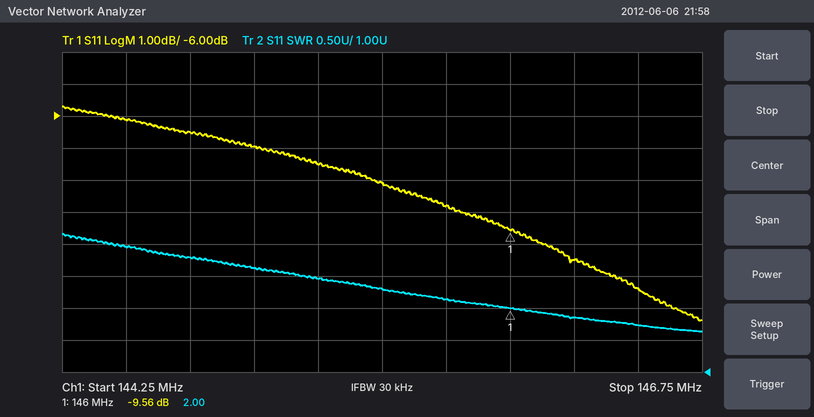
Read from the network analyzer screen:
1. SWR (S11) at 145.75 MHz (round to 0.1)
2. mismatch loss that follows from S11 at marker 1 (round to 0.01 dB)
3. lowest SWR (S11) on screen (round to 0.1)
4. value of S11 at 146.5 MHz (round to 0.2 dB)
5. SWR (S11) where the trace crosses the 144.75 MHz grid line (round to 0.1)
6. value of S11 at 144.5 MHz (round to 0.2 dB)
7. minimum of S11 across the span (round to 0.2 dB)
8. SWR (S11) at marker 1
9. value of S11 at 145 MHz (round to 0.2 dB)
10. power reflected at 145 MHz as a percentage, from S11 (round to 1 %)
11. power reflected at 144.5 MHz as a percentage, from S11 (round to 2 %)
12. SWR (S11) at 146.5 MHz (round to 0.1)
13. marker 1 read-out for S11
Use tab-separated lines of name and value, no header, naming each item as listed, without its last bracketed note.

SWR (S11) at 145.75 MHz	2.1
mismatch loss that follows from S11 at marker 1	0.51 dB
lowest SWR (S11) on screen	1.6
value of S11 at 146.5 MHz	-11.4 dB
SWR (S11) where the trace crosses the 144.75 MHz grid line	2.8
value of S11 at 144.5 MHz	-6.2 dB
minimum of S11 across the span	-12.4 dB
SWR (S11) at marker 1	2.00
value of S11 at 145 MHz	-7.0 dB
power reflected at 145 MHz as a percentage, from S11	20 %
power reflected at 144.5 MHz as a percentage, from S11	24 %
SWR (S11) at 146.5 MHz	1.7
marker 1 read-out for S11	-9.56 dB
